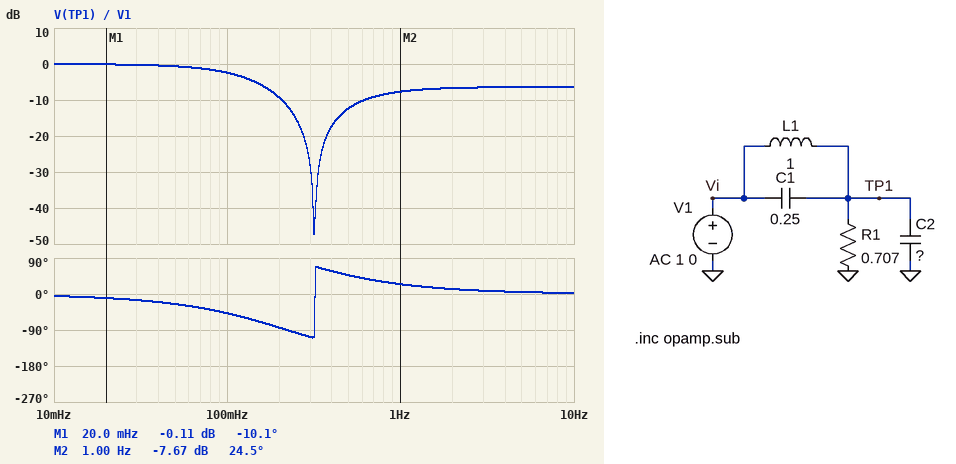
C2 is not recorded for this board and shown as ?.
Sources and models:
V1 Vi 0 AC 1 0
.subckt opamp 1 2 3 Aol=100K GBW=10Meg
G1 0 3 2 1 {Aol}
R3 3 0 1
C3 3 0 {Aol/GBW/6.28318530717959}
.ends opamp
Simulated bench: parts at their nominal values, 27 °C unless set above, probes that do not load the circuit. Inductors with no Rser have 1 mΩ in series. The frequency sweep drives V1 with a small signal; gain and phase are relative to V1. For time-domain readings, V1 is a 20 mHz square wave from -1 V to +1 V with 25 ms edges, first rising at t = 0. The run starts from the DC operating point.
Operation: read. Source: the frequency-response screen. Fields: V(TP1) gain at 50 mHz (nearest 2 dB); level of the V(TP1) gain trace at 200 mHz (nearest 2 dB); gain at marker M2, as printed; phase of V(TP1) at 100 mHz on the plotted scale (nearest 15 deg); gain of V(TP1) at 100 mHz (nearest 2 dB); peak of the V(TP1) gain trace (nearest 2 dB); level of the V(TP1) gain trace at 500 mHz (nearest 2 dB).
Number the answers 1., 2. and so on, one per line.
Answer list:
1. 0 dB
2. -10 dB
3. -7.67 dB
4. -45 deg
5. -2 dB
6. 0 dB
7. -12 dB
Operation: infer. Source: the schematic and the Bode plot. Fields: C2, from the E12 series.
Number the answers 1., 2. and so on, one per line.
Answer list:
1. 270 mF
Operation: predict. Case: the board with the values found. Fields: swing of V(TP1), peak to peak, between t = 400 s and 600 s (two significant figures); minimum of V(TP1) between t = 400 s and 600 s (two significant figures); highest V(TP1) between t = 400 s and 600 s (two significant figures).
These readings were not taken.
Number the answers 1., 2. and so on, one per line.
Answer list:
1. 2.0 V
2. -1.0 V
3. 1.0 V
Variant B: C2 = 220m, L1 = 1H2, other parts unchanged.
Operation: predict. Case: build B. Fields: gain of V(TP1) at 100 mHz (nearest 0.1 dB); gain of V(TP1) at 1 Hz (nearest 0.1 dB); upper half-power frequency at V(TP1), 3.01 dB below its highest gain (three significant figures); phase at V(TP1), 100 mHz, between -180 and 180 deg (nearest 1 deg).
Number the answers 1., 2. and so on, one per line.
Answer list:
1. -3.5 dB
2. -6.8 dB
3. 92.0 mHz
4. -54 deg
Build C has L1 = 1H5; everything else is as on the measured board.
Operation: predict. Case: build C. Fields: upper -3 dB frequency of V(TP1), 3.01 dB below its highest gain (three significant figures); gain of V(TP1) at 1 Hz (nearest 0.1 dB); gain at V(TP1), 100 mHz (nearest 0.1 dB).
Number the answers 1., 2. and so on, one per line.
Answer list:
1. 75.0 mHz
2. -7.5 dB
3. -4.9 dB
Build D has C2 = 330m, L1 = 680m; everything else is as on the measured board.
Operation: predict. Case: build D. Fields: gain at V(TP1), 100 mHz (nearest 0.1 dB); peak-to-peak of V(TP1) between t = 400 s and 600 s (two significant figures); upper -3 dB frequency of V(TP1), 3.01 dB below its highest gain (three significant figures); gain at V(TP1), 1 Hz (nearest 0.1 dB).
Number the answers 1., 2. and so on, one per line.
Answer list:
1. -0.9 dB
2. 2.1 V
3. 166 mHz
4. -8.8 dB
